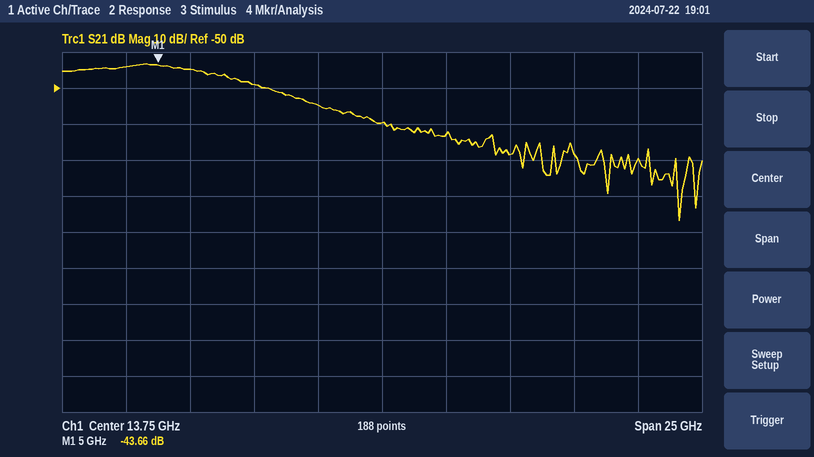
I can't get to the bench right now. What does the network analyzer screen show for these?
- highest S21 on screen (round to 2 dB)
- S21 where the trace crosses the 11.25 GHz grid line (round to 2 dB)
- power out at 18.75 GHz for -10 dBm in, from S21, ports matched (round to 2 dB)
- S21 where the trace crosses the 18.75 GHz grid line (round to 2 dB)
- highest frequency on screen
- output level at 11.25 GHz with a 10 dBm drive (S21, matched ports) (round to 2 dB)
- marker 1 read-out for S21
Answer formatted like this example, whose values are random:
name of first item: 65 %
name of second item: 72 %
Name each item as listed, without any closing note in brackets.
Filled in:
highest S21 on screen: -44 dB
S21 where the trace crosses the 11.25 GHz grid line: -54 dB
power out at 18.75 GHz for -10 dBm in, from S21, ports matched: -78 dBm
S21 where the trace crosses the 18.75 GHz grid line: -68 dB
highest frequency on screen: 26.25 GHz
output level at 11.25 GHz with a 10 dBm drive (S21, matched ports): -44 dBm
marker 1 read-out for S21: -43.66 dB
